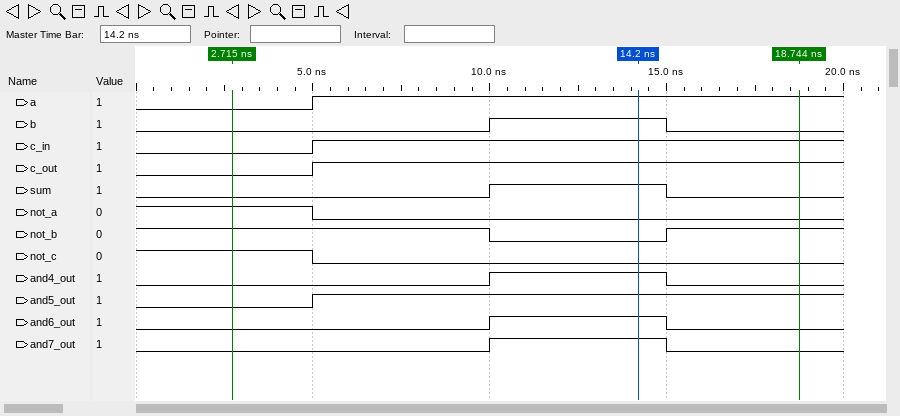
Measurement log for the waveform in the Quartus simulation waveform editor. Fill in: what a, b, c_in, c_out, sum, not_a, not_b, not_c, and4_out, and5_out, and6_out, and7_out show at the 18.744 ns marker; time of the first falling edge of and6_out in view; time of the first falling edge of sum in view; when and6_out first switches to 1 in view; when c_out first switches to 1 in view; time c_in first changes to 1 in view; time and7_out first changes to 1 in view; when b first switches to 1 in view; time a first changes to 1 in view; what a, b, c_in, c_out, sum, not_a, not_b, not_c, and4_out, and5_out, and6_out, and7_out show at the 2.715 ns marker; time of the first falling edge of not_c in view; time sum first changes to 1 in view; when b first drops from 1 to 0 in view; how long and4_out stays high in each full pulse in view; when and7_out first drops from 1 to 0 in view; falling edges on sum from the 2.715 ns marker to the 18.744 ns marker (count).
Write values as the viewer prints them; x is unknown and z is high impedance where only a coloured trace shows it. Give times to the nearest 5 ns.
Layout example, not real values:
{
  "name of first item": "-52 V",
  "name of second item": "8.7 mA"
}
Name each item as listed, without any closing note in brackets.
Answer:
{
  "what a, b, c_in, c_out, sum, not_a, not_b, not_c, and4_out, and5_out, and6_out, and7_out show at the 18.744 ns marker": "a=1, b=0, c_in=1, c_out=1, sum=0, not_a=0, not_b=1, not_c=0, and4_out=0, and5_out=1, and6_out=0, and7_out=0",
  "time of the first falling edge of and6_out in view": "15 ns",
  "time of the first falling edge of sum in view": "15 ns",
  "when and6_out first switches to 1 in view": "10 ns",
  "when c_out first switches to 1 in view": "5 ns",
  "time c_in first changes to 1 in view": "5 ns",
  "time and7_out first changes to 1 in view": "10 ns",
  "when b first switches to 1 in view": "10 ns",
  "time a first changes to 1 in view": "5 ns",
  "what a, b, c_in, c_out, sum, not_a, not_b, not_c, and4_out, and5_out, and6_out, and7_out show at the 2.715 ns marker": "a=0, b=0, c_in=0, c_out=0, sum=0, not_a=1, not_b=1, not_c=1, and4_out=0, and5_out=0, and6_out=0, and7_out=0",
  "time of the first falling edge of not_c in view": "5 ns",
  "time sum first changes to 1 in view": "10 ns",
  "when b first drops from 1 to 0 in view": "15 ns",
  "how long and4_out stays high in each full pulse in view": "5 ns",
  "when and7_out first drops from 1 to 0 in view": "15 ns",
  "falling edges on sum from the 2.715 ns marker to the 18.744 ns marker": "1"
}
